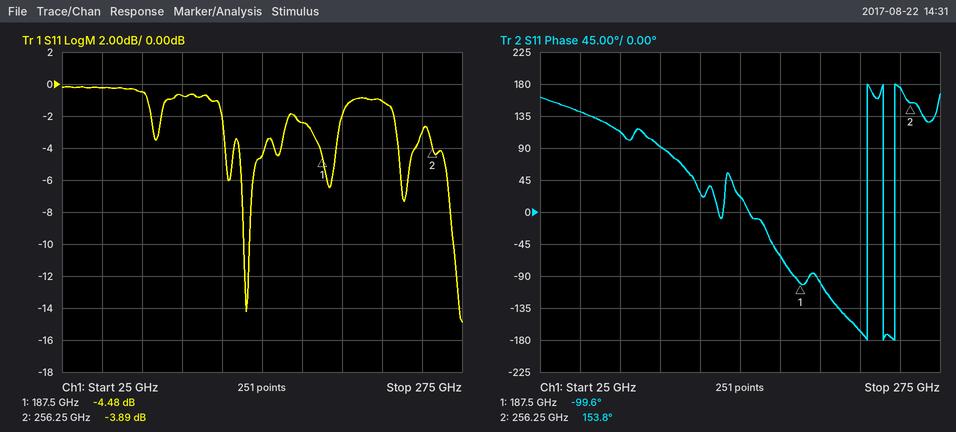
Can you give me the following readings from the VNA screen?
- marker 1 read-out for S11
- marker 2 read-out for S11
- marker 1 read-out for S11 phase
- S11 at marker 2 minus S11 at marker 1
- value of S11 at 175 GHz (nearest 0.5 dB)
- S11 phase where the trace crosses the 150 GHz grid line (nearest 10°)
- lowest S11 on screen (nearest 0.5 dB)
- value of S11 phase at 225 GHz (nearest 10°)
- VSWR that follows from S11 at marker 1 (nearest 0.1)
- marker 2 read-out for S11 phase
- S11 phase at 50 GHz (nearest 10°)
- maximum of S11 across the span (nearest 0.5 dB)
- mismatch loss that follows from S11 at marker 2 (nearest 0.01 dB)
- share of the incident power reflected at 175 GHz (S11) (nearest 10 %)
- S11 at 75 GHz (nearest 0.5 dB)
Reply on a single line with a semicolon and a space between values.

-4.48 dB; -3.89 dB; -99.6°; 0.59 dB; -2.5 dB; 20°; -15.0 dB; -170°; 4.0; 153.8°; 140°; 0.0 dB; 2.28 dB; 60 %; -0.5 dB
